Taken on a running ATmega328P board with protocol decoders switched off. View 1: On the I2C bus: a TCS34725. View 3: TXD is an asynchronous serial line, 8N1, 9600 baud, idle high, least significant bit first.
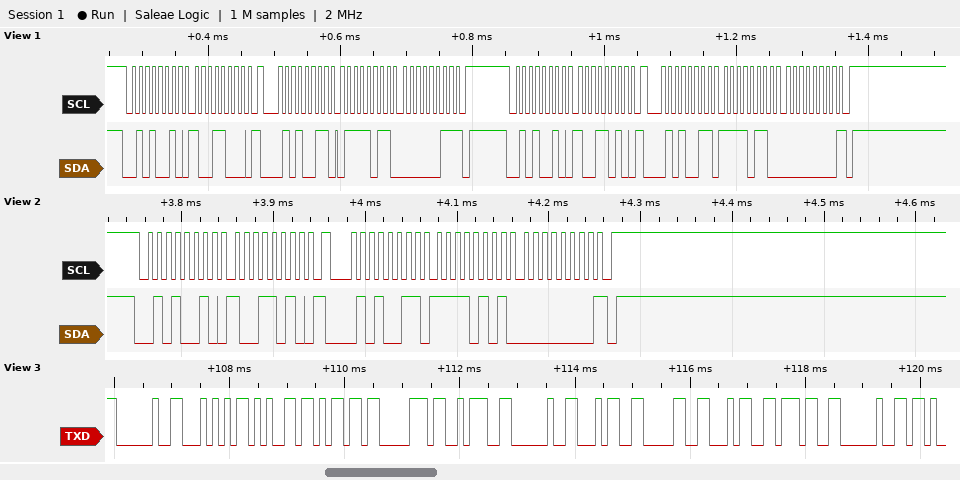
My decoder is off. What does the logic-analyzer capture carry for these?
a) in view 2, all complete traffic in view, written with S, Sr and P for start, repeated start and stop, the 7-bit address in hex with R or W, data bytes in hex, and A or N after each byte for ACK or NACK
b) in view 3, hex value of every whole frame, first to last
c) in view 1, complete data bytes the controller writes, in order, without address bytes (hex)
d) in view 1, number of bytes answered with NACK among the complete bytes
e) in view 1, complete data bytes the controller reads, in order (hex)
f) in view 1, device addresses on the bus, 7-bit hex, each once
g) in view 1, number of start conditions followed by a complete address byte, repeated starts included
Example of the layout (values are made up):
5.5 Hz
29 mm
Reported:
S 29W A 9A A Sr 29R A F5 A 00 N P
0x20 0x54 0x65 0x6D 0x70 0x3A 0x20 0x34 0x30 0x34 0x37 0x20
98 9A
2
7B 03 F6 00
0x29
4
